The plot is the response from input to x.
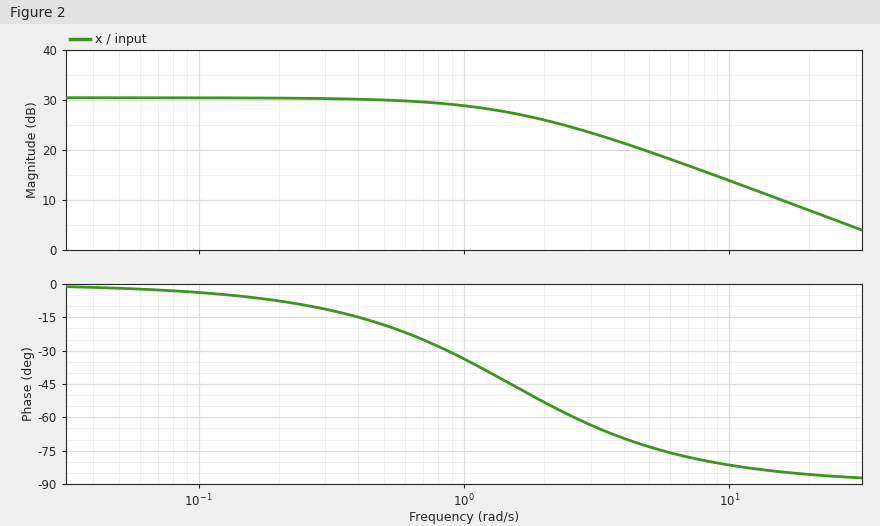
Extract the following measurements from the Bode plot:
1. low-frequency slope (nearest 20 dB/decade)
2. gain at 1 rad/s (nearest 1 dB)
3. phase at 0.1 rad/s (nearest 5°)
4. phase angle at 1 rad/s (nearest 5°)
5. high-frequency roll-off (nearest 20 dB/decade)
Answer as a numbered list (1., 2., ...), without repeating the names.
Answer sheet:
1. 0 dB/decade
2. 29 dB
3. -5°
4. -35°
5. -20 dB/decade
